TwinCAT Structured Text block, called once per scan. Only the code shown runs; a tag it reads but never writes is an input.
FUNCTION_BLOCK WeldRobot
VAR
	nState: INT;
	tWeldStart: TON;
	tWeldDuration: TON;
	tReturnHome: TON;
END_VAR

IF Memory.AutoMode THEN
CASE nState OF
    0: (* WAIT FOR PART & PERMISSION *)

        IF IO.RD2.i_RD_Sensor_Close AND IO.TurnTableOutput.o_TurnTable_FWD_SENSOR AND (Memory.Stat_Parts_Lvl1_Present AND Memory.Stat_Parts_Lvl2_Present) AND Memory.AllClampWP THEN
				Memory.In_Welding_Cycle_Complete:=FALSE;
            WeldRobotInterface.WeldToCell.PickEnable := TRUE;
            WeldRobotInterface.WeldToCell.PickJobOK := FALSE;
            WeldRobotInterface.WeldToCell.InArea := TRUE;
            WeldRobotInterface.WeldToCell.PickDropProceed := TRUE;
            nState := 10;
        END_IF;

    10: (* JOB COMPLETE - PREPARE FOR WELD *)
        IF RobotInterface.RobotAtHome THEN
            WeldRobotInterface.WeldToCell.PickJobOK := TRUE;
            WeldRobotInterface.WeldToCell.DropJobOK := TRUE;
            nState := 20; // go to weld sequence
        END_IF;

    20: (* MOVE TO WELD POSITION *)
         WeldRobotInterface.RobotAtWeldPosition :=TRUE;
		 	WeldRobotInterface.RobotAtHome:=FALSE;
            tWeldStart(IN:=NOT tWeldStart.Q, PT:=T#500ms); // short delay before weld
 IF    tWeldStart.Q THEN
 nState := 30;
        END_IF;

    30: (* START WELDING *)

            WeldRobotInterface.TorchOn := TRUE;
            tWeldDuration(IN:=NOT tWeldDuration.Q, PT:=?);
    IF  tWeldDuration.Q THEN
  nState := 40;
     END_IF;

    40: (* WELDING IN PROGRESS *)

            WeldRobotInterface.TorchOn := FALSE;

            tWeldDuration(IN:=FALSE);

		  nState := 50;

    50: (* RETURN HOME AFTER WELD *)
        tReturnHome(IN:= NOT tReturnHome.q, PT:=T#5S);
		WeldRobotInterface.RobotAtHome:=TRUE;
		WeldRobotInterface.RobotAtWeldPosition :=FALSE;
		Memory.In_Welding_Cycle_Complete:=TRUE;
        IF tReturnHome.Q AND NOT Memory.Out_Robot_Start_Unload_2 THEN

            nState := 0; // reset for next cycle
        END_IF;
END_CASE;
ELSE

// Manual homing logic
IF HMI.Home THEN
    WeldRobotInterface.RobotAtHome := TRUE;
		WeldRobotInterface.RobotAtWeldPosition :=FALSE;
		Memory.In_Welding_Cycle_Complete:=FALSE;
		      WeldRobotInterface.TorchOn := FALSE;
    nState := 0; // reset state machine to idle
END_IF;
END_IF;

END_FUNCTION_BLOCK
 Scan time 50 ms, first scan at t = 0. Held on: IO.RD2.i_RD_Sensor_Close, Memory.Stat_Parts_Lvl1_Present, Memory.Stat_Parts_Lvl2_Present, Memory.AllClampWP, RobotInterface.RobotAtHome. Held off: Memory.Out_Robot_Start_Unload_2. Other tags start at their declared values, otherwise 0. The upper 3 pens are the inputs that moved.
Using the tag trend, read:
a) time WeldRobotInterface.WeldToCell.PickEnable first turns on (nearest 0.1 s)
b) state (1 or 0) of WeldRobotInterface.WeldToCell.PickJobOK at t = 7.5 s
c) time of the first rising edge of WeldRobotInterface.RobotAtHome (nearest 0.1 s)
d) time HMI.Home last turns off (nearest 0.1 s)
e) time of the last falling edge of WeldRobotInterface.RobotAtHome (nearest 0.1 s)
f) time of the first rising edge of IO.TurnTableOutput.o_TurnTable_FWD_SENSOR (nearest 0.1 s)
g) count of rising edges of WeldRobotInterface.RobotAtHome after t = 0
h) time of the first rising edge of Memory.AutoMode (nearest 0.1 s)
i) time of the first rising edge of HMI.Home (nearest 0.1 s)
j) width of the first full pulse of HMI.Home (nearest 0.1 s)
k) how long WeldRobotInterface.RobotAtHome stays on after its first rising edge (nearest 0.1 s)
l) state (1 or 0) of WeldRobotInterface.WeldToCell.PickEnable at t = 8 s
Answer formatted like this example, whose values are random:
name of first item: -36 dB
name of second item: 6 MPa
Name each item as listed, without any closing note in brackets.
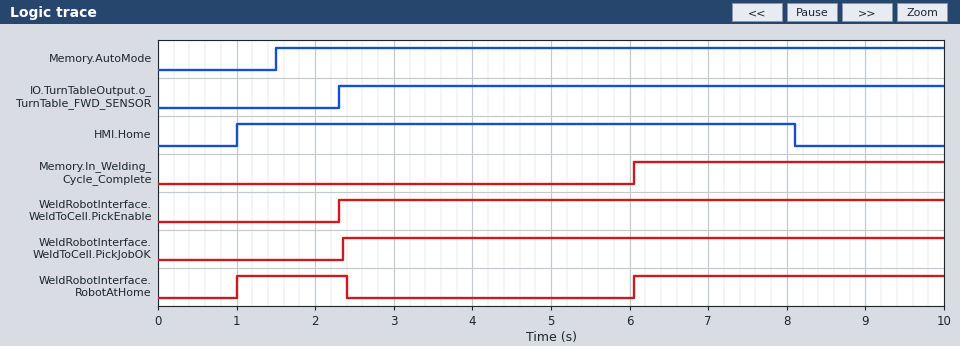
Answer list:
time WeldRobotInterface.WeldToCell.PickEnable first turns on: 2.3 s
state (1 or 0) of WeldRobotInterface.WeldToCell.PickJobOK at t = 7.5 s: 1
time of the first rising edge of WeldRobotInterface.RobotAtHome: 1.0 s
time HMI.Home last turns off: 8.1 s
time of the last falling edge of WeldRobotInterface.RobotAtHome: 2.4 s
time of the first rising edge of IO.TurnTableOutput.o_TurnTable_FWD_SENSOR: 2.3 s
count of rising edges of WeldRobotInterface.RobotAtHome after t = 0: 2
time of the first rising edge of Memory.AutoMode: 1.5 s
time of the first rising edge of HMI.Home: 1.0 s
width of the first full pulse of HMI.Home: 7.1 s
how long WeldRobotInterface.RobotAtHome stays on after its first rising edge: 1.4 s
state (1 or 0) of WeldRobotInterface.WeldToCell.PickEnable at t = 8 s: 1
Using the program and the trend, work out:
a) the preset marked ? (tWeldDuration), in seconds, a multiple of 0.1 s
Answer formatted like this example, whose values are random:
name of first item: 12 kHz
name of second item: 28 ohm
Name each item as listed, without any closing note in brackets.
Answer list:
the preset marked ? (tWeldDuration), in seconds, a multiple of 0.1 s: 3.0 s
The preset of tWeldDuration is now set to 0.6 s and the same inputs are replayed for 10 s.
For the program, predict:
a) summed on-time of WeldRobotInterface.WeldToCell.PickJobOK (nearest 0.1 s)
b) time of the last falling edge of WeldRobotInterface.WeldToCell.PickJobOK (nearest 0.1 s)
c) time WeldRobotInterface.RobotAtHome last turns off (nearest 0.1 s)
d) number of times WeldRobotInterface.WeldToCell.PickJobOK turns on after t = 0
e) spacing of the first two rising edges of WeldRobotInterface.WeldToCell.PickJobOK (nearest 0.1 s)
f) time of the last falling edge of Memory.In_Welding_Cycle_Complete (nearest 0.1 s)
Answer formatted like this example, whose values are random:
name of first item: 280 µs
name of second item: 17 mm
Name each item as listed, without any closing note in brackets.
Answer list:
summed on-time of WeldRobotInterface.WeldToCell.PickJobOK: 7.6 s
time of the last falling edge of WeldRobotInterface.WeldToCell.PickJobOK: 8.7 s
time WeldRobotInterface.RobotAtHome last turns off: 8.8 s
number of times WeldRobotInterface.WeldToCell.PickJobOK turns on after t = 0: 2
spacing of the first two rising edges of WeldRobotInterface.WeldToCell.PickJobOK: 6.4 s
time of the last falling edge of Memory.In_Welding_Cycle_Complete: 8.7 s
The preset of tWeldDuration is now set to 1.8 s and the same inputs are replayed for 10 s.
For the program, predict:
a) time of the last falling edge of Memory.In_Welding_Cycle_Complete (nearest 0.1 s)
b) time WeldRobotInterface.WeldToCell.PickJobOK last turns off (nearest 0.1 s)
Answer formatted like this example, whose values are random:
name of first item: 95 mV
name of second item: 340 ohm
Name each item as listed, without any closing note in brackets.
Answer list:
time of the last falling edge of Memory.In_Welding_Cycle_Complete: 9.9 s
time WeldRobotInterface.WeldToCell.PickJobOK last turns off: 9.9 s
